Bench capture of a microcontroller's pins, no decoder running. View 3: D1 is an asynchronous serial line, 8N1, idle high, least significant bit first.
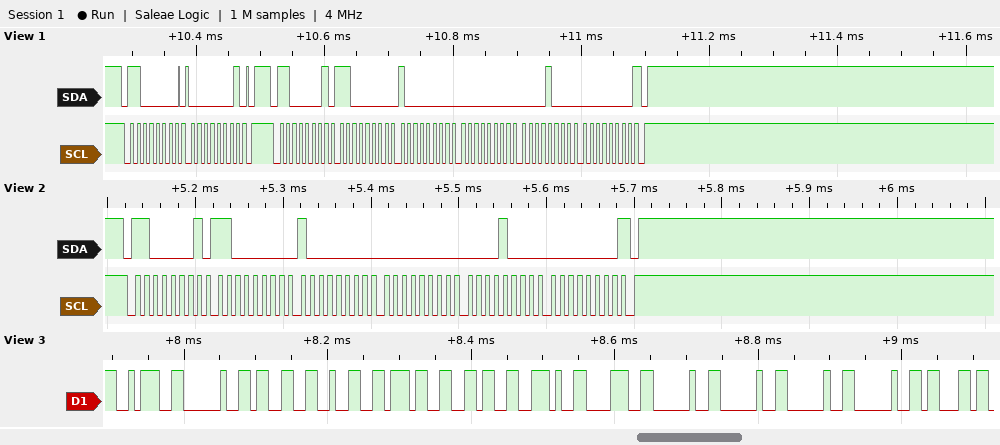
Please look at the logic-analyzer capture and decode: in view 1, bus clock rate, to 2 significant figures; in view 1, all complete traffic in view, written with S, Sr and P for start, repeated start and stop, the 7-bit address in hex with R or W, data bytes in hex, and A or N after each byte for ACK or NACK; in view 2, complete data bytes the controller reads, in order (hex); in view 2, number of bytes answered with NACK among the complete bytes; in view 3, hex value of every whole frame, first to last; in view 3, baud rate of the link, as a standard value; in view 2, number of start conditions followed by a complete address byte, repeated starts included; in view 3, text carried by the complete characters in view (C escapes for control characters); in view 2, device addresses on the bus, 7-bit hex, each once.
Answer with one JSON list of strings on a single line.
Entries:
["100 kHz", "S 60W A 01 A P S 60R A C0 A 80 A 00 A 08 A 00 N P", "C0 80 00 08 00", "1", "0x3A 0x20 0x33 0x32 0x37 0x36 0x2E 0x38 0x20 0x20 0x20 0x20 0x63", "115200 baud", "1", "\": 3276.8    c\"", "0x60"]
